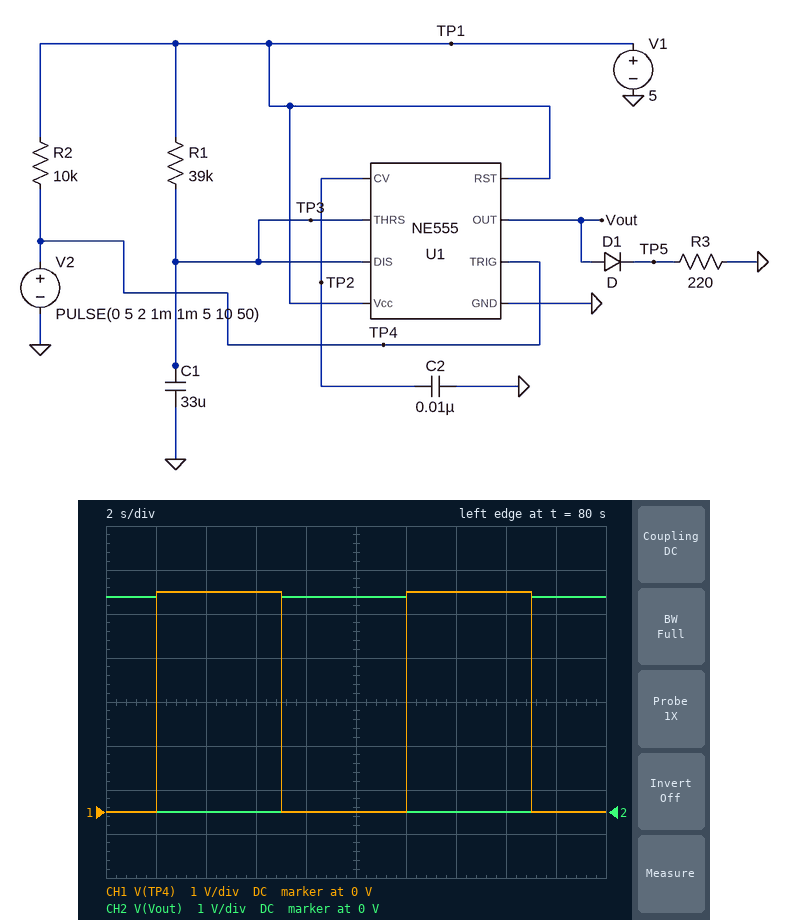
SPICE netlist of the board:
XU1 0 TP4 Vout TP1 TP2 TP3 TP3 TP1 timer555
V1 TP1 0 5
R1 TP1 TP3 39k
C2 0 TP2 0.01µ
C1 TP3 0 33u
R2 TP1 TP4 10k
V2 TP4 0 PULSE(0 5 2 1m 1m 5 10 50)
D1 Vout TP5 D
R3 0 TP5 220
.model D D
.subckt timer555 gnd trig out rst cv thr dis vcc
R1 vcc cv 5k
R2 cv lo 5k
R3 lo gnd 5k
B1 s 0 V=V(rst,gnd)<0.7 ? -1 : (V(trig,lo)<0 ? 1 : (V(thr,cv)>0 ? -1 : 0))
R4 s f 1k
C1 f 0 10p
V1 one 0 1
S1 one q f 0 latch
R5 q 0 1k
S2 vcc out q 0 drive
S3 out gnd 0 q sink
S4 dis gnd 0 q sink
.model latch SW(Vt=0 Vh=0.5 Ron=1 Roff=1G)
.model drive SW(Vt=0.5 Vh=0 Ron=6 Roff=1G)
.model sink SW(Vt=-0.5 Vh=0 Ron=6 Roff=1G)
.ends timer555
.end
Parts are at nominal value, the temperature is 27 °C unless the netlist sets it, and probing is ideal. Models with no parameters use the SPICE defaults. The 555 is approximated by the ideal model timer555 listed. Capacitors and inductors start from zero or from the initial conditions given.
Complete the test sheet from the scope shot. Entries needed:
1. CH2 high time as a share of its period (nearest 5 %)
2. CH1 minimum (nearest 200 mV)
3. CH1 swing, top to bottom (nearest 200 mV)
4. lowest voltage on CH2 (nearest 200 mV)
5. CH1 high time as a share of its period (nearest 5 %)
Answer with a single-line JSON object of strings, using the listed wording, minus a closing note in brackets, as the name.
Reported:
{"CH2 high time as a share of its period": "50 %", "CH1 minimum": "0 V", "CH1 swing, top to bottom": "5.0 V", "lowest voltage on CH2": "0 V", "CH1 high time as a share of its period": "50 %"}
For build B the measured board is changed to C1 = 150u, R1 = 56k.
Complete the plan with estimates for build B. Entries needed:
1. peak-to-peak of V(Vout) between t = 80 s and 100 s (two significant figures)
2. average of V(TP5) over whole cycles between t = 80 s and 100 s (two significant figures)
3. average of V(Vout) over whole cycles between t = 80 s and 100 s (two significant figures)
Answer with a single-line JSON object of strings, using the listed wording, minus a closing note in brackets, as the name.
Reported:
{"peak-to-peak of V(Vout) between t = 80 s and 100 s": "4.9 V", "average of V(TP5) over whole cycles between t = 80 s and 100 s": "3.8 V", "average of V(Vout) over whole cycles between t = 80 s and 100 s": "4.5 V"}
